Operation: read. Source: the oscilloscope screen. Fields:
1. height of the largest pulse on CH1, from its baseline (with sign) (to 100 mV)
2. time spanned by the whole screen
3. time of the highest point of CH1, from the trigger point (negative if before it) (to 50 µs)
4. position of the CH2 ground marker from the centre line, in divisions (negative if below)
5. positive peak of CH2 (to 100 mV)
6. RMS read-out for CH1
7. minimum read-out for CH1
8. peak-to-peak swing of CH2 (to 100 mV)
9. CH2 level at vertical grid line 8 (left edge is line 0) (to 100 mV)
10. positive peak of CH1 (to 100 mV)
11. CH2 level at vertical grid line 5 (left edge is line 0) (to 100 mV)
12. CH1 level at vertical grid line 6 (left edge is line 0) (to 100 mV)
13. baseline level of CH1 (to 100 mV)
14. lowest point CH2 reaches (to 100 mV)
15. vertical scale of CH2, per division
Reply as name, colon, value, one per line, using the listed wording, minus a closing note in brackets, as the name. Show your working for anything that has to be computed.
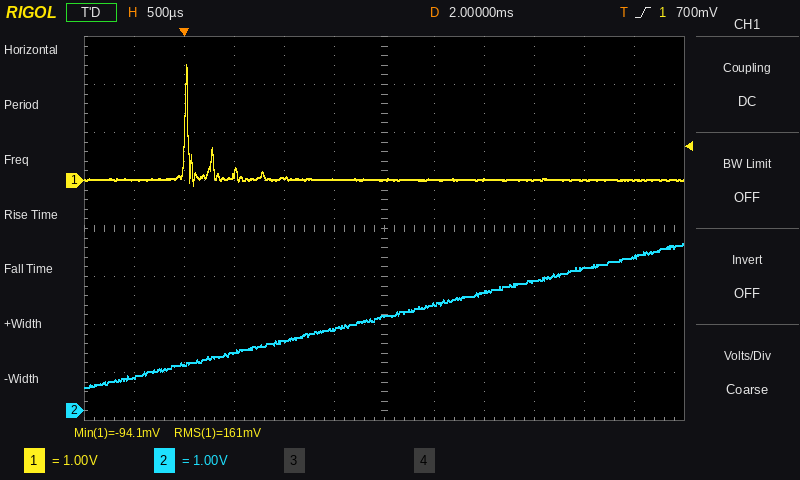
height of the largest pulse on CH1, from its baseline (with sign): 2.4 V − (0.0 V) = +2.4 V
time spanned by the whole screen: 6 ms
time of the highest point of CH1, from the trigger point (negative if before it): +50 µs
position of the CH2 ground marker from the centre line, in divisions: -3.8 div
positive peak of CH2: 3.5 V
RMS read-out for CH1: 161 mV
minimum read-out for CH1: -94.1 mV
peak-to-peak swing of CH2: 3.5 V − (500 mV) = 3.0 V
CH2 level at vertical grid line 8 (left edge is line 0): 2.5 V
positive peak of CH1: 2.4 V
CH2 level at vertical grid line 5 (left edge is line 0): 1.7 V
CH1 level at vertical grid line 6 (left edge is line 0): 0.0 V
baseline level of CH1: 0.0 V
lowest point CH2 reaches: 500 mV
vertical scale of CH2, per division: 1 V
